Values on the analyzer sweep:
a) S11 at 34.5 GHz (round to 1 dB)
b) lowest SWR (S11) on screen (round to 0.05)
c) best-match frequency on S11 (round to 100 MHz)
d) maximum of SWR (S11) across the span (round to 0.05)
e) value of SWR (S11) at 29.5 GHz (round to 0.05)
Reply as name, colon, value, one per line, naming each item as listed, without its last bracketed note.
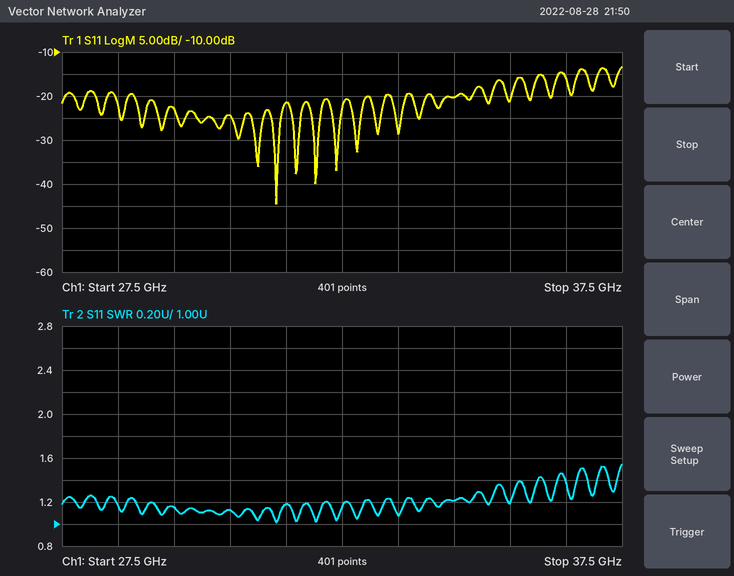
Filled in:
S11 at 34.5 GHz: -20 dB
lowest SWR (S11) on screen: 1.00
best-match frequency on S11: 31.3 GHz
maximum of SWR (S11) across the span: 1.55
value of SWR (S11) at 29.5 GHz: 1.15
